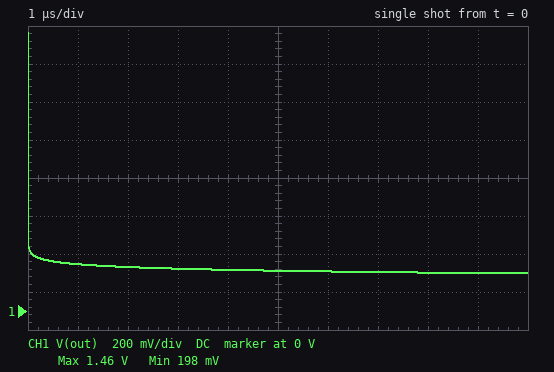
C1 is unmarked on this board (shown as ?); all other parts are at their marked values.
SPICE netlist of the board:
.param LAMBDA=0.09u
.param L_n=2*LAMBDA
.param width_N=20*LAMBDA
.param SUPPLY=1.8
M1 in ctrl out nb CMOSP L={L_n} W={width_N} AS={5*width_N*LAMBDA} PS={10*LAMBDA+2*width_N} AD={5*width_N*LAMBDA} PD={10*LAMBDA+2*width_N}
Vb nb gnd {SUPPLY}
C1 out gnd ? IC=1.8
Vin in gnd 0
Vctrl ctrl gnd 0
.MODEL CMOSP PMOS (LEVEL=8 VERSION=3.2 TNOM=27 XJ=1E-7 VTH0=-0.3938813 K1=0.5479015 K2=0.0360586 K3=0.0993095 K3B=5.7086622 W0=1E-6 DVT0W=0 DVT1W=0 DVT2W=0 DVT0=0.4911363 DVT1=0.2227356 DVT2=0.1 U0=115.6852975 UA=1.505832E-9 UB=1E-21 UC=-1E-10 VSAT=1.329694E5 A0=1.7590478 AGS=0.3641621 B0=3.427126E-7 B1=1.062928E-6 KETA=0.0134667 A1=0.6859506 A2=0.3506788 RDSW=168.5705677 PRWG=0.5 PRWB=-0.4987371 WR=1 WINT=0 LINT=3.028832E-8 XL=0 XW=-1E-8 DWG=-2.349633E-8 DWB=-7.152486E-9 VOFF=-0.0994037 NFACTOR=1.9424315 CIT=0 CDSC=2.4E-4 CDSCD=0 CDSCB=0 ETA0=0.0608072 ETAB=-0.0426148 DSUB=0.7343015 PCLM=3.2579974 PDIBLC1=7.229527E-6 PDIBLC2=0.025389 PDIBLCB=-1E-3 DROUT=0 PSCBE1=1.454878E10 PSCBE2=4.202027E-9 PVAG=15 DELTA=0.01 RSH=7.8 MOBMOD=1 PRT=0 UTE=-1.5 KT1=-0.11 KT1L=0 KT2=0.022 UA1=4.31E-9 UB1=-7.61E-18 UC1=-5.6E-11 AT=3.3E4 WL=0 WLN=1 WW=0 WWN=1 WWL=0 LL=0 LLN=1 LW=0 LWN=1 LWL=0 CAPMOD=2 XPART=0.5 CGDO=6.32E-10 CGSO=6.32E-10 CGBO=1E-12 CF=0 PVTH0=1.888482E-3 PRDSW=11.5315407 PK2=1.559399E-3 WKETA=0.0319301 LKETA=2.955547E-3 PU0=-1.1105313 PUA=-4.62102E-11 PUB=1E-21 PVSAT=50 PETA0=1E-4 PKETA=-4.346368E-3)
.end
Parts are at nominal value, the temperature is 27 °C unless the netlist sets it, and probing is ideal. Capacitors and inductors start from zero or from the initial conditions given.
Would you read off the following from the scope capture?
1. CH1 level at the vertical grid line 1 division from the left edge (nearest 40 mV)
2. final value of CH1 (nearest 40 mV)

240 mV
200 mV
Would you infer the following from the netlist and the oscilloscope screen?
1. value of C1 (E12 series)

47 pF
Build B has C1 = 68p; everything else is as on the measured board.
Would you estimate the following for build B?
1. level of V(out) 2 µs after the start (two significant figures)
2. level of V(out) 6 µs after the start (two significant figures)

240 mV
220 mV
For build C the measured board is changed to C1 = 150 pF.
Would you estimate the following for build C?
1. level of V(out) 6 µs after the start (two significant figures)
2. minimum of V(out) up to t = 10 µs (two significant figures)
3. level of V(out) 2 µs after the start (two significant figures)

230 mV
220 mV
260 mV
